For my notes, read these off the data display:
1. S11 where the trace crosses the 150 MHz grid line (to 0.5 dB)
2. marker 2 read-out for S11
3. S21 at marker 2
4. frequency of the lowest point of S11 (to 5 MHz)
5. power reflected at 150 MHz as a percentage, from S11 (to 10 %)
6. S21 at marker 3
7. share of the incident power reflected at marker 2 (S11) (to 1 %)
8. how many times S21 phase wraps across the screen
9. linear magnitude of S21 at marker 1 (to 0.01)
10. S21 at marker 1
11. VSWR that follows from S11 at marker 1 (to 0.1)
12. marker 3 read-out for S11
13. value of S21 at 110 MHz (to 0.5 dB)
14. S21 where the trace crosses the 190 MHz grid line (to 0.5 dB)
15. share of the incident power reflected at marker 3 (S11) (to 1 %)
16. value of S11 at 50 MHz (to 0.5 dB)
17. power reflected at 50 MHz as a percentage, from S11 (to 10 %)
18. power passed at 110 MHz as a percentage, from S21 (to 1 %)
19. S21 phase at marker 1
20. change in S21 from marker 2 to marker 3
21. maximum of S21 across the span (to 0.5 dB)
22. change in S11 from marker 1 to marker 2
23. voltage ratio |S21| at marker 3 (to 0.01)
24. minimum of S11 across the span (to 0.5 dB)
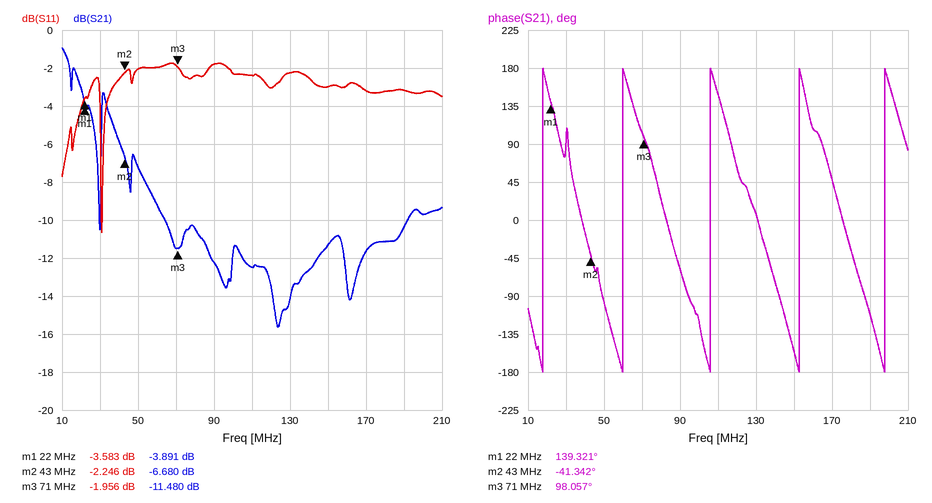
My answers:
-3.0 dB
-2.246 dB
-6.680 dB
30 MHz
50 %
-11.480 dB
60 %
5
0.64
-3.891 dB
4.9
-1.956 dB
-12.5 dB
-10.5 dB
64 %
-2.0 dB
60 %
6 %
139.321°
-4.800 dB
-1.0 dB
1.337 dB
0.27
-10.5 dB
